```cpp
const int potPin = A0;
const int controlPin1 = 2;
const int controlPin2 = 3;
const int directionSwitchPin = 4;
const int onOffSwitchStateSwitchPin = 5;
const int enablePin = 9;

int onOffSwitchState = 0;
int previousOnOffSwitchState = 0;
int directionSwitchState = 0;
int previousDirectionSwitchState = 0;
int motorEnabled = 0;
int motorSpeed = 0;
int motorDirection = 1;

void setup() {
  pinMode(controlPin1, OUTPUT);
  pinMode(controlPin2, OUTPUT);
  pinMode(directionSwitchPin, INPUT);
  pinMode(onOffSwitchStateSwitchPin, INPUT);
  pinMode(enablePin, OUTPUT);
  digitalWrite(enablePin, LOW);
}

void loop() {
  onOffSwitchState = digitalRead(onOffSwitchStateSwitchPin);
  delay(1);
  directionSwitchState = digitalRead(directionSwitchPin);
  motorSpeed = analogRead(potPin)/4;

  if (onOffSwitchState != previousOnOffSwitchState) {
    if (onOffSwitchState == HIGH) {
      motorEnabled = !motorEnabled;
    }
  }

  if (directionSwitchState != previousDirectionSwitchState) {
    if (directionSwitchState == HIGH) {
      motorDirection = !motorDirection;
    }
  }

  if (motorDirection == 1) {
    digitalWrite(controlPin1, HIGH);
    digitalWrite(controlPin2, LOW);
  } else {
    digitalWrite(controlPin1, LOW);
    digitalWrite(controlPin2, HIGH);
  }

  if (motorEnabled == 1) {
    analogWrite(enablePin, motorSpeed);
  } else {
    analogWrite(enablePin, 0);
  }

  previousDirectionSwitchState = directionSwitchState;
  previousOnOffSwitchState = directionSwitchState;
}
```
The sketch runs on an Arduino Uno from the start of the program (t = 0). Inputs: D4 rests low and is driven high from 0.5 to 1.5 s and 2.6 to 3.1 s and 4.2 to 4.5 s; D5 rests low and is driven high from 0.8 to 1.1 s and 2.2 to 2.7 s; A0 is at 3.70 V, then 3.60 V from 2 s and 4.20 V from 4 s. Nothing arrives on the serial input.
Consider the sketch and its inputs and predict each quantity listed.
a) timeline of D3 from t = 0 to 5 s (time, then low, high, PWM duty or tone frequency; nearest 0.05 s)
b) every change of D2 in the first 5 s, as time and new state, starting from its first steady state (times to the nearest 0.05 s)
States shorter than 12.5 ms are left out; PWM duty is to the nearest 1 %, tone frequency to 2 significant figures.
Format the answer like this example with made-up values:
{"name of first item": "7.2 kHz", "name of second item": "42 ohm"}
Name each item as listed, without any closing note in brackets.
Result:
{"timeline of D3 from t = 0 to 5 s": "0 s low; 0.5 s high; 2.6 s low; 4.2 s high", "every change of D2 in the first 5 s, as time and new state, starting from its first steady state": "0 s high; 0.5 s low; 2.6 s high; 4.2 s low"}
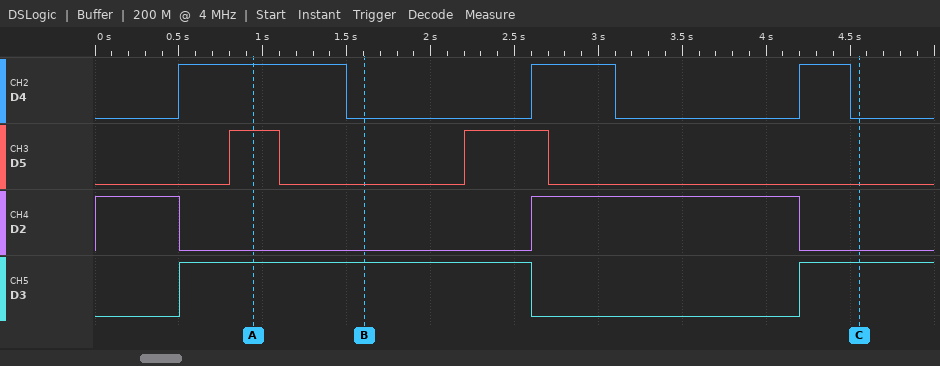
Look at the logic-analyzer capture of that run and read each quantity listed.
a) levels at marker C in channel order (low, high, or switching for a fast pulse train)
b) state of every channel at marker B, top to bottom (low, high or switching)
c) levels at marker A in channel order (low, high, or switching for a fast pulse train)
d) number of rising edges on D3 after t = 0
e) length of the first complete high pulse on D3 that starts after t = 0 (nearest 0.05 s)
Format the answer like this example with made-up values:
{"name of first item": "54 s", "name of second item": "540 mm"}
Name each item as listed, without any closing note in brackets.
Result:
{"levels at marker C in channel order": "D4 low, D5 low, D2 low, D3 high", "state of every channel at marker B, top to bottom": "D4 low, D5 low, D2 low, D3 high", "levels at marker A in channel order": "D4 high, D5 high, D2 low, D3 high", "number of rising edges on D3 after t = 0": "2", "length of the first complete high pulse on D3 that starts after t = 0": "2.10 s"}
